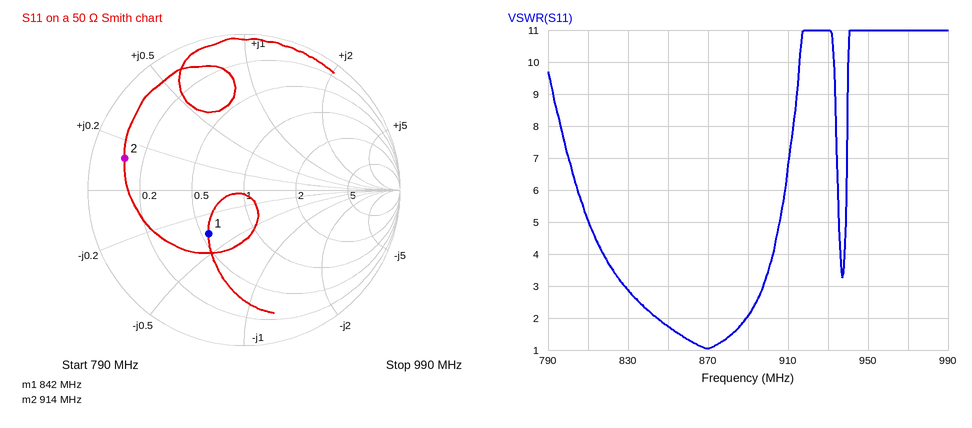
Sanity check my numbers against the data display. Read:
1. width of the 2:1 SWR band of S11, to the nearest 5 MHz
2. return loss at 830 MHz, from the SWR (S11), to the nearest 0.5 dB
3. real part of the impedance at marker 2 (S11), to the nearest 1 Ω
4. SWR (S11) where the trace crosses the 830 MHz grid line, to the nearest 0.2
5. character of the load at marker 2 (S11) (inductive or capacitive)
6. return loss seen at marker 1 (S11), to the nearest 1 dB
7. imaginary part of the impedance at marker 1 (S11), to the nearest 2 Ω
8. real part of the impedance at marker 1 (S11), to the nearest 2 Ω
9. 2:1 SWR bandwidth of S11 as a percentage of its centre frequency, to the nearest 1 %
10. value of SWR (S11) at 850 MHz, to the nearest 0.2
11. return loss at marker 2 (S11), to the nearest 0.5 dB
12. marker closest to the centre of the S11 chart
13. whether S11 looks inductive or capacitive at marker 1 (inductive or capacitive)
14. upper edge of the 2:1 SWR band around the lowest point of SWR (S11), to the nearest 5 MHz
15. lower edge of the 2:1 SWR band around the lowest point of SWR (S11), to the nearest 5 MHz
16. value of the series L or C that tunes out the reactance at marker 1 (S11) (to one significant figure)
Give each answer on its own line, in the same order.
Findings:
45 MHz
6.5 dB
6 Ω
2.8
inductive
9 dB
-18 Ω
28 Ω
5 %
1.8
2.0 dB
marker 1
capacitive
890 MHz
845 MHz
3 nH
